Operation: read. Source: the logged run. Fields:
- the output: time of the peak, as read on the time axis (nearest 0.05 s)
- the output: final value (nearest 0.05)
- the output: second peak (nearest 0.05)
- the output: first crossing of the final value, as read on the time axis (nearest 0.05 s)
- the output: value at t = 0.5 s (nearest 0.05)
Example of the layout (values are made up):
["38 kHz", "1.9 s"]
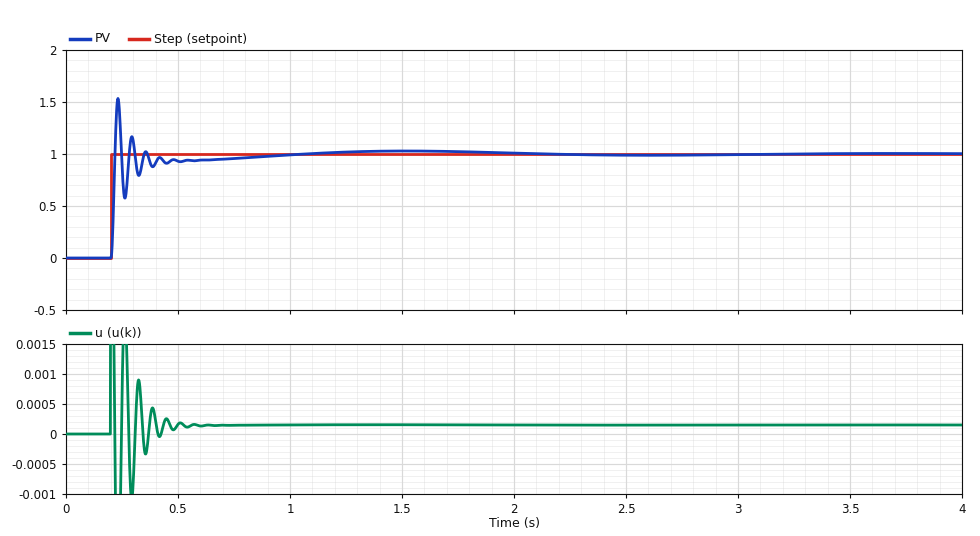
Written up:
["0.25 s", "1.00", "1.15", "0.20 s", "0.95"]
